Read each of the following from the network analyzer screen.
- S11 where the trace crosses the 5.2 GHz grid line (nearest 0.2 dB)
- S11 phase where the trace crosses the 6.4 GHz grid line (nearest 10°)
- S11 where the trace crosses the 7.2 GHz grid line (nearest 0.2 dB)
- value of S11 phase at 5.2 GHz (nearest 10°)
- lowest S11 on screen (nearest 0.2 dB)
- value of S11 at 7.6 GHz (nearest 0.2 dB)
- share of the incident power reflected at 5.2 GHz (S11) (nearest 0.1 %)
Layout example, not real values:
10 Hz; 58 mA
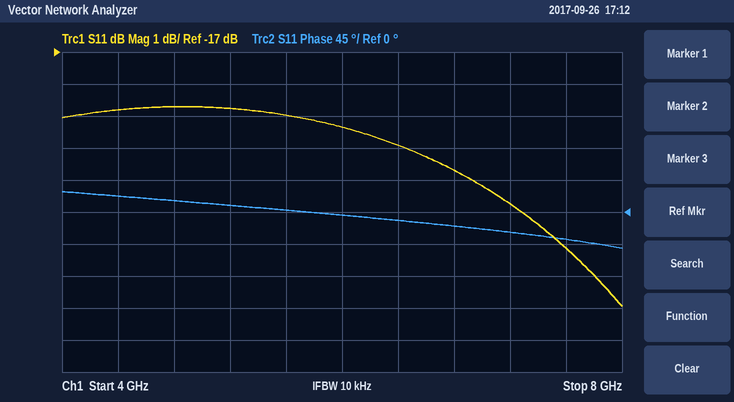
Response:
-18.8 dB; -10°; -21.8 dB; 10°; -25.0 dB; -23.2 dB; 1.3 %
